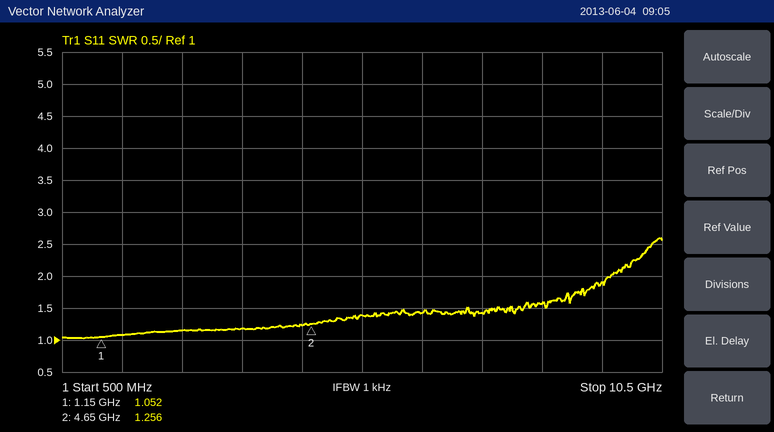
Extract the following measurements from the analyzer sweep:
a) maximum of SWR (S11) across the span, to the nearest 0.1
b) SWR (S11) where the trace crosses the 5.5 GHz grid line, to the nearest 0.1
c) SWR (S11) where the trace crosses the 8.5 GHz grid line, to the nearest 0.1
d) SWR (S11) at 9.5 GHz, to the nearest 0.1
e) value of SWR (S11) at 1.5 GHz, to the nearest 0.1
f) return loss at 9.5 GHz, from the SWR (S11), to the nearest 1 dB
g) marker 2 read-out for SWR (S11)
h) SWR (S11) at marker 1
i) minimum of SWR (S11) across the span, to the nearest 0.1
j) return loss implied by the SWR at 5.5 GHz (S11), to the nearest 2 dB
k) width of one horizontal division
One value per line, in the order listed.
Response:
2.6
1.4
1.6
1.9
1.1
10 dB
1.256
1.052
1.0
16 dB
1 GHz
